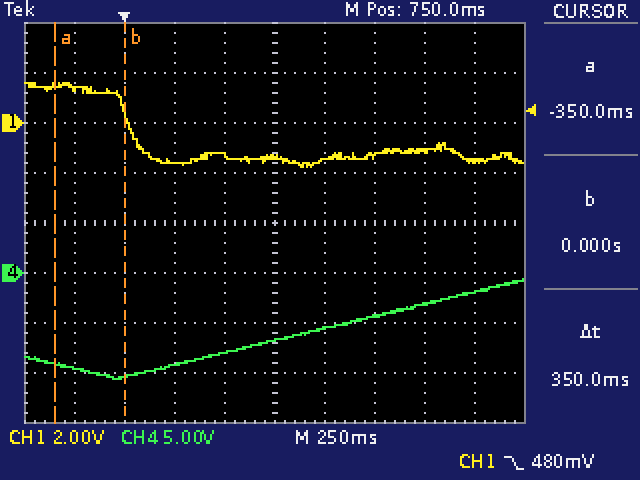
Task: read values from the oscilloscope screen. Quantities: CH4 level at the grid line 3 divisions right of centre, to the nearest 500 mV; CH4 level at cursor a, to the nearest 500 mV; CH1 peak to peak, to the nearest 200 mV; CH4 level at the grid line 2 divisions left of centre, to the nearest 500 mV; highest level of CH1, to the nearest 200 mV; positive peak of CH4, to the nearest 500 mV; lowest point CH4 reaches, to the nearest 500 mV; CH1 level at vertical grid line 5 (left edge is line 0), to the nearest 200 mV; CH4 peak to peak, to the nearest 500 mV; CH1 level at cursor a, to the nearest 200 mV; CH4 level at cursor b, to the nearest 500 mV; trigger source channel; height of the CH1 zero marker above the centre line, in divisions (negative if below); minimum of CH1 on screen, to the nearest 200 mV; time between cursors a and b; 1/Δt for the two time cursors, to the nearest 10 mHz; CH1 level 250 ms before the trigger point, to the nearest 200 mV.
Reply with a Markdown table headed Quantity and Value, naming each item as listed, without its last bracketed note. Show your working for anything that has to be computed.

| Quantity | Value |
|---|---|
| CH4 level at the grid line 3 divisions right of centre, to the nearest 500 mV | -3.0 V |
| CH4 level at cursor a, to the nearest 500 mV | -9.0 V |
| CH1 peak to peak, to the nearest 200 mV | 1.6 V − (-1.8 V) = 3.4 V |
| CH4 level at the grid line 2 divisions left of centre, to the nearest 500 mV | -9.0 V |
| highest level of CH1, to the nearest 200 mV | 1.6 V |
| positive peak of CH4, to the nearest 500 mV | -500 mV |
| lowest point CH4 reaches, to the nearest 500 mV | -10.5 V |
| CH1 level at vertical grid line 5 (left edge is line 0), to the nearest 200 mV | -1.4 V |
| CH4 peak to peak, to the nearest 500 mV | -500 mV − (-10.5 V) = 10.0 V |
| CH1 level at cursor a, to the nearest 200 mV | 1.4 V |
| CH4 level at cursor b, to the nearest 500 mV | -10.5 V |
| trigger source channel | CH1 |
| height of the CH1 zero marker above the centre line, in divisions | +2.0 div |
| minimum of CH1 on screen, to the nearest 200 mV | -1.8 V |
| time between cursors a and b | 350 ms |
| 1/Δt for the two time cursors, to the nearest 10 mHz | 1 / 350 ms ≈ 2.86 Hz |
| CH1 level 250 ms before the trigger point, to the nearest 200 mV | 1.4 V |
